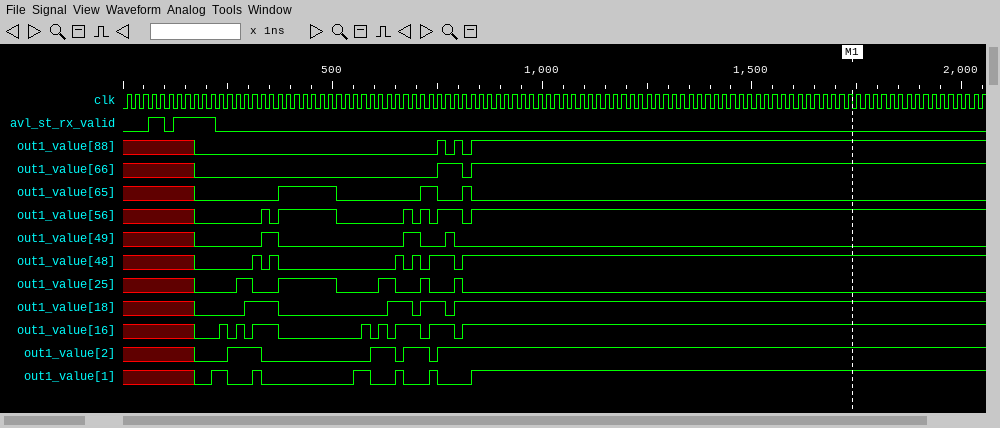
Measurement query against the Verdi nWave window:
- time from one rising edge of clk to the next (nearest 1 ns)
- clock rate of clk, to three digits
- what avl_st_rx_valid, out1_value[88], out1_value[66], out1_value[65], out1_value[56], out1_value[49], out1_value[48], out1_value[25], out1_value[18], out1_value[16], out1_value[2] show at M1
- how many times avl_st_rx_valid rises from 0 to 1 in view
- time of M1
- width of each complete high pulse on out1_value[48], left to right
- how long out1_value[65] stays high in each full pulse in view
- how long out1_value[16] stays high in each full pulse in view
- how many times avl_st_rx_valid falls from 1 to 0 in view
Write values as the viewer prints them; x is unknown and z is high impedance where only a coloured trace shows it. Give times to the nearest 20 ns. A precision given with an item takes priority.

20 ns
50.0 MHz
avl_st_rx_valid=0, out1_value[88]=1, out1_value[66]=1, out1_value[65]=0, out1_value[56]=1, out1_value[49]=0, out1_value[48]=1, out1_value[25]=0, out1_value[18]=1, out1_value[16]=1, out1_value[2]=1
2
1740 ns
20 ns, 20 ns, 20 ns, 20 ns, 60 ns
140 ns, 40 ns, 20 ns
20 ns, 20 ns, 60 ns, 20 ns, 20 ns, 60 ns, 60 ns
2
